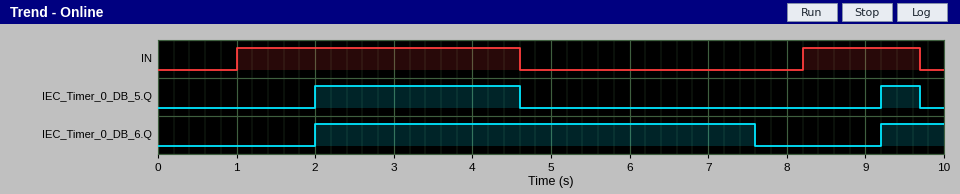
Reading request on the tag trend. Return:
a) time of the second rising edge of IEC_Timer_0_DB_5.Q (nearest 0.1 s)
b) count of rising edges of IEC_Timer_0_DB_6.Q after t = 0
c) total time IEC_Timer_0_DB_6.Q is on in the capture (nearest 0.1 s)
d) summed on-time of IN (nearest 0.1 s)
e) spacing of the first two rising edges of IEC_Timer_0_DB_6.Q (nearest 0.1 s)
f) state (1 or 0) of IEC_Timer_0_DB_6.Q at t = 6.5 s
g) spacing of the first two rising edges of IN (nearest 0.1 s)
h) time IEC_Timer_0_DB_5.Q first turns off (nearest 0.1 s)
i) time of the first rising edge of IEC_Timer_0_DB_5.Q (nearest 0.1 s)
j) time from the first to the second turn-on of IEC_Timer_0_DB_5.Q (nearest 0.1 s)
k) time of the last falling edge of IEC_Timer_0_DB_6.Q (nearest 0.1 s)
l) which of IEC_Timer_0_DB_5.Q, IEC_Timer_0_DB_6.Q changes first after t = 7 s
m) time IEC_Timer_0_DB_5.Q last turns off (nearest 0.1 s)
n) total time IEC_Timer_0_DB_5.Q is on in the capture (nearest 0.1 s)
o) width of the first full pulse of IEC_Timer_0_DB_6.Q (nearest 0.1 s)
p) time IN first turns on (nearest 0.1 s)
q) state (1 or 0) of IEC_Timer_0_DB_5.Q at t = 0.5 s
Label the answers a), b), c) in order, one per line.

a) 9.2 s
b) 2
c) 6.4 s
d) 5.1 s
e) 7.2 s
f) 1
g) 7.2 s
h) 4.6 s
i) 2.0 s
j) 7.2 s
k) 7.6 s
l) IEC_Timer_0_DB_6.Q
m) 9.7 s
n) 3.1 s
o) 5.6 s
p) 1.0 s
q) 0
